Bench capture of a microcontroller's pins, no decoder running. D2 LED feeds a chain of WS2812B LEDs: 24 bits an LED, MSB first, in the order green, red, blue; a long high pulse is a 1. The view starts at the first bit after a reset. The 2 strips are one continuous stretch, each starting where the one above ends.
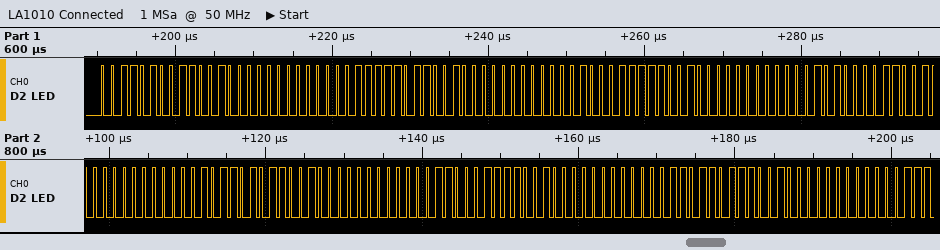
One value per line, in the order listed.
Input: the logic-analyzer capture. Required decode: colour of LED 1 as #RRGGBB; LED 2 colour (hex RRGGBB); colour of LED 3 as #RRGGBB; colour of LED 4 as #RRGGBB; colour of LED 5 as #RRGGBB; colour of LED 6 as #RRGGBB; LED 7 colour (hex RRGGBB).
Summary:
#C83400
#C83E00
#C84700
#C85000
#C85A00
#C86300
#C86D00
